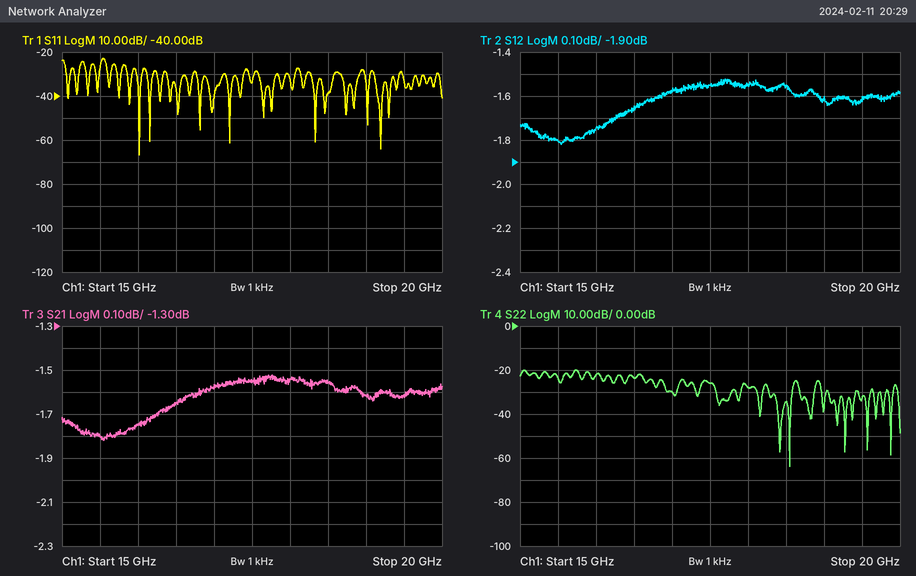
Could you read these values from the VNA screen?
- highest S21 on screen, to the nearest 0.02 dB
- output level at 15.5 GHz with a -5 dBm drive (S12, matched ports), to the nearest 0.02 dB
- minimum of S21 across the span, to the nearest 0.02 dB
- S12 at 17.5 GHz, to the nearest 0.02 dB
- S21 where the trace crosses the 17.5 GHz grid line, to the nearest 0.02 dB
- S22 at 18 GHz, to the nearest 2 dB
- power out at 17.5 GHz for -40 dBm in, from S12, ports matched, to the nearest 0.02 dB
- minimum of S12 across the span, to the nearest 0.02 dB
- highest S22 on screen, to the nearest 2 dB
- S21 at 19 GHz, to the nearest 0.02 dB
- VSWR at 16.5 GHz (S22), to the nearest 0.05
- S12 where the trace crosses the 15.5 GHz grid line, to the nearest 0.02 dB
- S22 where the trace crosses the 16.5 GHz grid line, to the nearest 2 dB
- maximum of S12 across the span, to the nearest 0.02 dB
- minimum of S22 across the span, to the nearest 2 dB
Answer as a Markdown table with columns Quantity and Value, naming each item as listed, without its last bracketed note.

| Quantity | Value |
|---|---|
| highest S21 on screen, to the nearest 0.02 dB | -1.52 dB |
| output level at 15.5 GHz with a -5 dBm drive (S12, matched ports), to the nearest 0.02 dB | -6.80 dBm |
| minimum of S21 across the span, to the nearest 0.02 dB | -1.82 dB |
| S12 at 17.5 GHz, to the nearest 0.02 dB | -1.56 dB |
| S21 where the trace crosses the 17.5 GHz grid line, to the nearest 0.02 dB | -1.56 dB |
| S22 at 18 GHz, to the nearest 2 dB | -28 dB |
| power out at 17.5 GHz for -40 dBm in, from S12, ports matched, to the nearest 0.02 dB | -41.56 dBm |
| minimum of S12 across the span, to the nearest 0.02 dB | -1.82 dB |
| highest S22 on screen, to the nearest 2 dB | -20 dB |
| S21 at 19 GHz, to the nearest 0.02 dB | -1.62 dB |
| VSWR at 16.5 GHz (S22), to the nearest 0.05 | 1.15 |
| S12 where the trace crosses the 15.5 GHz grid line, to the nearest 0.02 dB | -1.80 dB |
| S22 where the trace crosses the 16.5 GHz grid line, to the nearest 2 dB | -24 dB |
| maximum of S12 across the span, to the nearest 0.02 dB | -1.52 dB |
| minimum of S22 across the span, to the nearest 2 dB | -64 dB |
